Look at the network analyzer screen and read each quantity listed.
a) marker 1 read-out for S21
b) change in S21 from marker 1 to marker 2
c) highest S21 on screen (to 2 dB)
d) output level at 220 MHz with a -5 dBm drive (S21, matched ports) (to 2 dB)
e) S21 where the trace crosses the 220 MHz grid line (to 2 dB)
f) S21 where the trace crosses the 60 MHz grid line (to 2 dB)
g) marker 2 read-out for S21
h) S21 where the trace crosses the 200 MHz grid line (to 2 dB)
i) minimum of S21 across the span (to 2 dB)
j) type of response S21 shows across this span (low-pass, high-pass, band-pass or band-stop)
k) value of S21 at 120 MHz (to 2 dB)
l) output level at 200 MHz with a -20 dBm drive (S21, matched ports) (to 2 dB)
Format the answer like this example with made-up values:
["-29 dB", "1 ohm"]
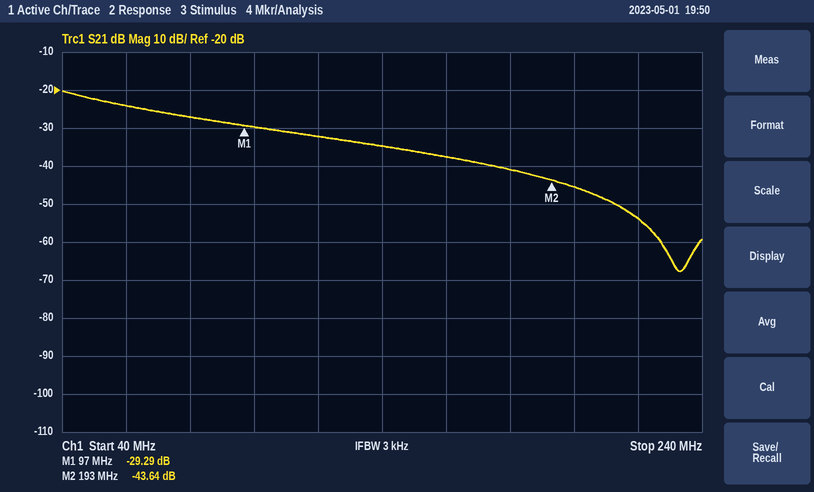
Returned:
["-29.29 dB", "-14.35 dB", "-20 dB", "-58 dBm", "-54 dB", "-24 dB", "-43.64 dB", "-46 dB", "-68 dB", "low-pass", "-32 dB", "-66 dBm"]
